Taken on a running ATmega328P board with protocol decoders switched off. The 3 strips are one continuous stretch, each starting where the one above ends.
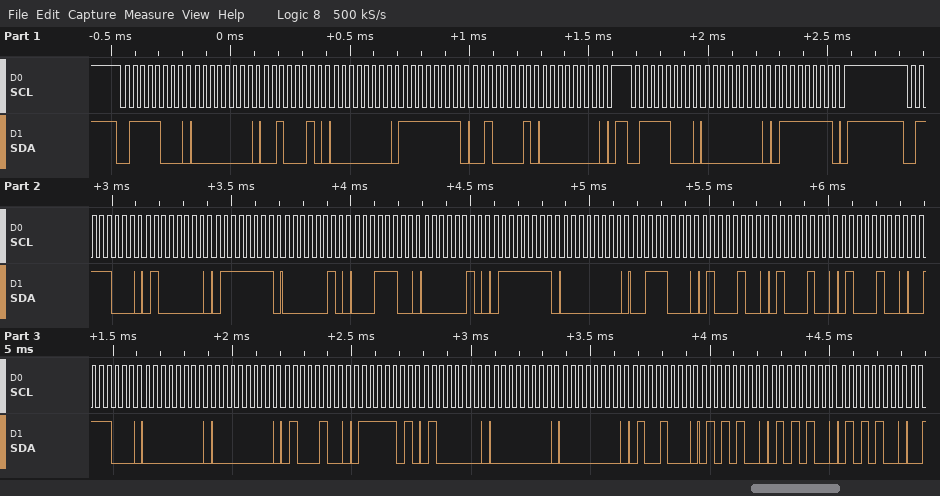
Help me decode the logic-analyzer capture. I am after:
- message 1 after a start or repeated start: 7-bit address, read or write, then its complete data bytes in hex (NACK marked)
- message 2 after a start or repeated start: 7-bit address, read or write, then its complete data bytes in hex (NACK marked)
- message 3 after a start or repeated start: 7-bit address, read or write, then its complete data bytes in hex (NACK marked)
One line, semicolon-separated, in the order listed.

0x3C write: 00 22 00 FF 21 00; 0x3C write: 00 7F; 0x3C write: 40 7F 02 1C 02 7F 00 38 44 44 44 38 00 00 44 7D 40 00 00 48 54 54 54
